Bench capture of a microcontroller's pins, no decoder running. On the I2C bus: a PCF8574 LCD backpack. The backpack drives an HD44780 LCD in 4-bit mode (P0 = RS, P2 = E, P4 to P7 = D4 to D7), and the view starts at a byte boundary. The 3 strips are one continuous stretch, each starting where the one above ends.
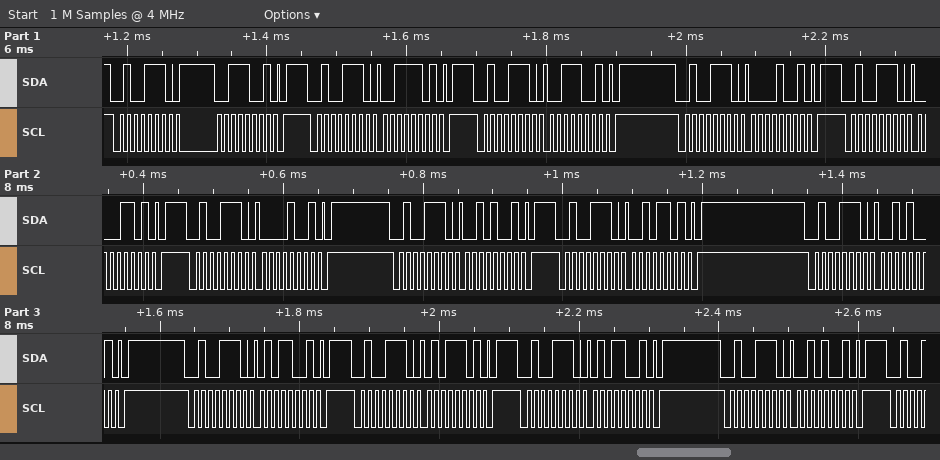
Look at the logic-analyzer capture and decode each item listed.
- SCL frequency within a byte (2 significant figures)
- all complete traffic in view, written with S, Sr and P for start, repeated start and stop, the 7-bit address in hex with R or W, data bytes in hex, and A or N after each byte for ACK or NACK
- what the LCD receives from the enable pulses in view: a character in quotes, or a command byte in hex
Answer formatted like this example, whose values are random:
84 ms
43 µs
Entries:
100 kHz
S 27W A 39 A P S 27W A 3D A P S 27W A 39 A P S 27W A 09 A P S 27W A 0D A P S 27W A 09 A P S 27W A 29 A P S 27W A 2D A P S 27W A 29 A P S 27W A 59 A P S 27W A 5D A P S 27W A 59 A P S 27W A 29 A P
'0' '%'
